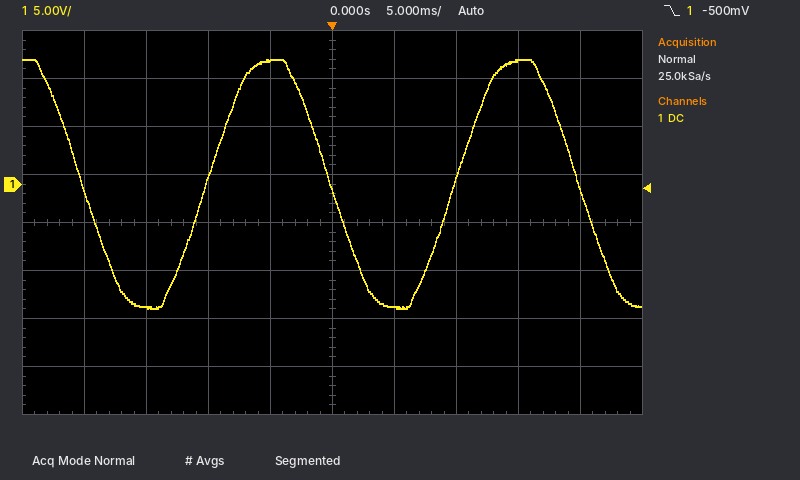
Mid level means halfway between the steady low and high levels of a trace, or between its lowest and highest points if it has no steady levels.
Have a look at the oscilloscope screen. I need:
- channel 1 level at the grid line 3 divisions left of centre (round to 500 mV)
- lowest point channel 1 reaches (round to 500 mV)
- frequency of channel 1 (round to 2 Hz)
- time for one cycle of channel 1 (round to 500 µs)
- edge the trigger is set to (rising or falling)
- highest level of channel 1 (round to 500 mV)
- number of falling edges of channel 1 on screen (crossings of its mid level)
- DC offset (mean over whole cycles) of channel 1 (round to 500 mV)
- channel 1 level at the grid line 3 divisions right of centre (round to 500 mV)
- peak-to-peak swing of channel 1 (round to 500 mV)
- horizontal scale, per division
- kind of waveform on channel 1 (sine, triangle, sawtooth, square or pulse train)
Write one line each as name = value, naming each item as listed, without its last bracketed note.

channel 1 level at the grid line 3 divisions left of centre = -13.0 V
lowest point channel 1 reaches = -13.0 V
frequency of channel 1 = 50 Hz
time for one cycle of channel 1 = 20.0 ms
edge the trigger is set to = falling
highest level of channel 1 = 13.0 V
number of falling edges of channel 1 on screen = 3
DC offset (mean over whole cycles) of channel 1 = 0.0 V
channel 1 level at the grid line 3 divisions right of centre = 13.0 V
peak-to-peak swing of channel 1 = 26.0 V
horizontal scale, per division = 5 ms
kind of waveform on channel 1 = sine
